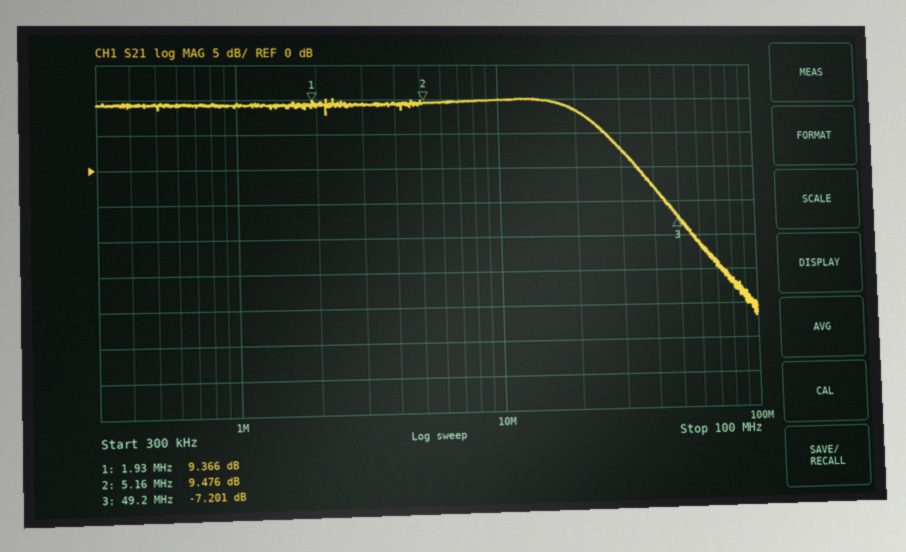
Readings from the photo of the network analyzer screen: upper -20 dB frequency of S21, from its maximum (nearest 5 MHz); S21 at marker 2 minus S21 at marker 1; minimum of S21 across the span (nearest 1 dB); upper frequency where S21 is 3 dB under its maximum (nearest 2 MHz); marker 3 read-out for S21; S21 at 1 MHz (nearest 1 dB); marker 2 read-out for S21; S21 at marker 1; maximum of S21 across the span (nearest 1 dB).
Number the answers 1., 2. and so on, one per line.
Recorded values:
1. 55 MHz
2. 0.110 dB
3. -22 dB
4. 22 MHz
5. -7.201 dB
6. 9 dB
7. 9.476 dB
8. 9.366 dB
9. 10 dB
